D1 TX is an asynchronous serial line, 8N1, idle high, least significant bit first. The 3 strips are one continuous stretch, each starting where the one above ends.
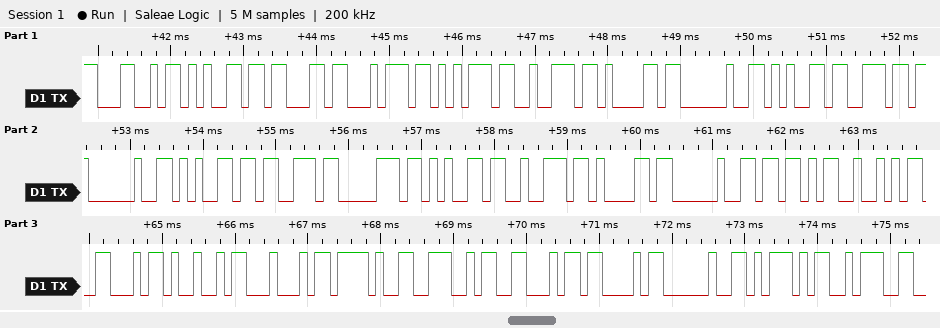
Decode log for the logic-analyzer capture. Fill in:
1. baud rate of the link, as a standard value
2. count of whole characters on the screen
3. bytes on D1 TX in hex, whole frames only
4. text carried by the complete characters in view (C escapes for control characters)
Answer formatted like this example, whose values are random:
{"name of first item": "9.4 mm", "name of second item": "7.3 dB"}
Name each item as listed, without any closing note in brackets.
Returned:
{"baud rate of the link, as a standard value": "9600 baud", "count of whole characters on the screen": "30", "bytes on D1 TX in hex, whole frames only": "0x4C 0x65 0x63 0x74 0x75 0x72 0x61 0x20 0x65 0x6E 0x20 0x65 0x73 0x70 0x65 0x72 0x61 0x20 0x5B 0x52 0x46 0x49 0x44 0x2F 0x4E 0x46 0x43 0x20 0x5D 0x3A", "text carried by the complete characters in view": "\"Lectura en espera [RFID/NFC ]:\""}
